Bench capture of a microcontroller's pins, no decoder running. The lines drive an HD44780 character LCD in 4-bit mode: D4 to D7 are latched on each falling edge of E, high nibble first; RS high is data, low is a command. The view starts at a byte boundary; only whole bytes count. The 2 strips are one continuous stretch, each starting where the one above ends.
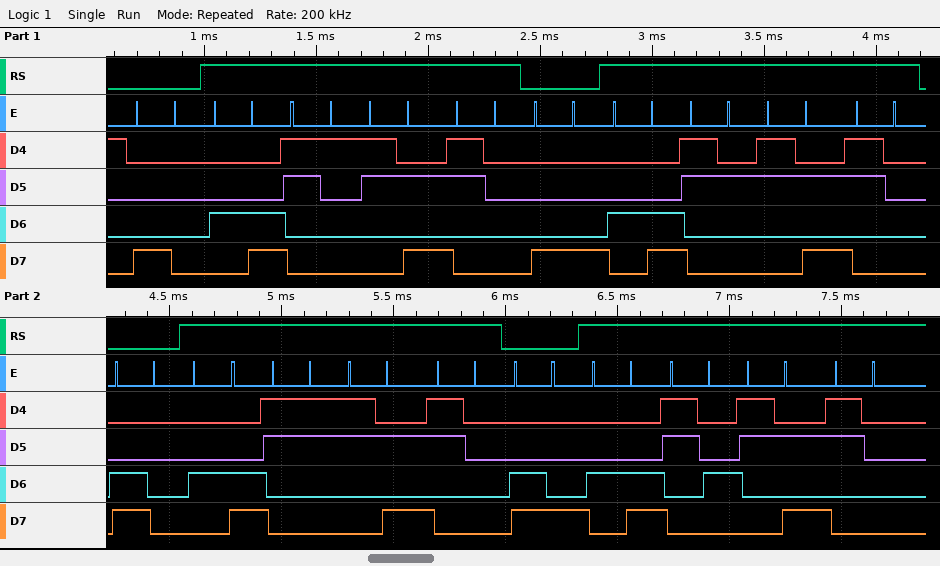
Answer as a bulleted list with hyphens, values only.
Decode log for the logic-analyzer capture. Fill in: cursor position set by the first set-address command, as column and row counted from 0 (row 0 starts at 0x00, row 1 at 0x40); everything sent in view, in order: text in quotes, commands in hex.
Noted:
- column 0, row 0
- 0x80 "L1:0" 0x88 "L2:0" 0xC0 "L3:0" 0xC8 "L4:0"
